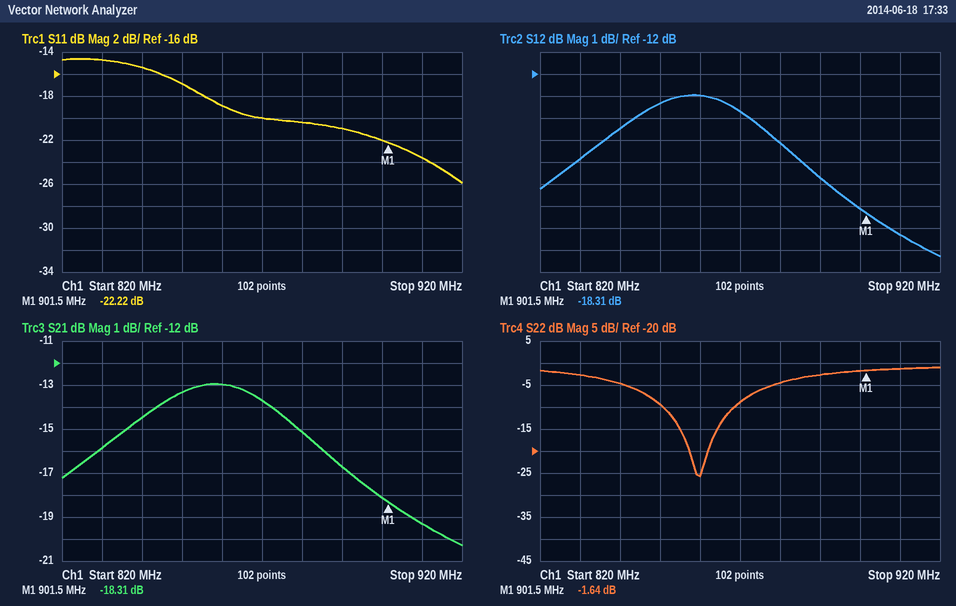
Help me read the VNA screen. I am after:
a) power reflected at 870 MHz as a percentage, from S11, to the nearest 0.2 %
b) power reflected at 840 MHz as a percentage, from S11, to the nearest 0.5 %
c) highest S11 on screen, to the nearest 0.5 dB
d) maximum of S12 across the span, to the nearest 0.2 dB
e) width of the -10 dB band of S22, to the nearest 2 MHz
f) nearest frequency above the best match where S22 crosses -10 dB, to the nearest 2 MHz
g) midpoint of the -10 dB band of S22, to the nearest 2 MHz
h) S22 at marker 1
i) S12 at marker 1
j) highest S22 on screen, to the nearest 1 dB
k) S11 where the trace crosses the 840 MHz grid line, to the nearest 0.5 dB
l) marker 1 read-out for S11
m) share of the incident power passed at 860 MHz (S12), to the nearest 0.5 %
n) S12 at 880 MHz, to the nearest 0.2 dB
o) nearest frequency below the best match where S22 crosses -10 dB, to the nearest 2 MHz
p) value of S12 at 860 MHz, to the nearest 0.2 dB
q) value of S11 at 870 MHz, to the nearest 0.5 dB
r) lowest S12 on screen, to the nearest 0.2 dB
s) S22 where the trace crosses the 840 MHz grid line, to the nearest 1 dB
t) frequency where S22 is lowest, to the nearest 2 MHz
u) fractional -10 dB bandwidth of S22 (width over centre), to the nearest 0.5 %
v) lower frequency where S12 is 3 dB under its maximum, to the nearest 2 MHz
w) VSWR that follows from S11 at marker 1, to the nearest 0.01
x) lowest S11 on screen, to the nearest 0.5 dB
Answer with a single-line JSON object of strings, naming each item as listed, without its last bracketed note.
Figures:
{"power reflected at 870 MHz as a percentage, from S11, to the nearest 0.2 %": "1.0 %", "power reflected at 840 MHz as a percentage, from S11, to the nearest 0.5 %": "3.0 %", "highest S11 on screen, to the nearest 0.5 dB": "-14.5 dB", "maximum of S12 across the span, to the nearest 0.2 dB": "-13.0 dB", "width of the -10 dB band of S22, to the nearest 2 MHz": "18 MHz", "nearest frequency above the best match where S22 crosses -10 dB, to the nearest 2 MHz": "868 MHz", "midpoint of the -10 dB band of S22, to the nearest 2 MHz": "860 MHz", "S22 at marker 1": "-1.64 dB", "S12 at marker 1": "-18.31 dB", "highest S22 on screen, to the nearest 1 dB": "-1 dB", "S11 where the trace crosses the 840 MHz grid line, to the nearest 0.5 dB": "-15.5 dB", "marker 1 read-out for S11": "-22.22 dB", "share of the incident power passed at 860 MHz (S12), to the nearest 0.5 %": "5.0 %", "S12 at 880 MHz, to the nearest 0.2 dB": "-15.2 dB", "nearest frequency below the best match where S22 crosses -10 dB, to the nearest 2 MHz": "850 MHz", "value of S12 at 860 MHz, to the nearest 0.2 dB": "-13.0 dB", "value of S11 at 870 MHz, to the nearest 0.5 dB": "-20.0 dB", "lowest S12 on screen, to the nearest 0.2 dB": "-20.2 dB", "S22 where the trace crosses the 840 MHz grid line, to the nearest 1 dB": "-5 dB", "frequency where S22 is lowest, to the nearest 2 MHz": "860 MHz", "fractional -10 dB bandwidth of S22 (width over centre), to the nearest 0.5 %": "2.0 %", "lower frequency where S12 is 3 dB under its maximum, to the nearest 2 MHz": "830 MHz", "VSWR that follows from S11 at marker 1, to the nearest 0.01": "1.17", "lowest S11 on screen, to the nearest 0.5 dB": "-26.0 dB"}
